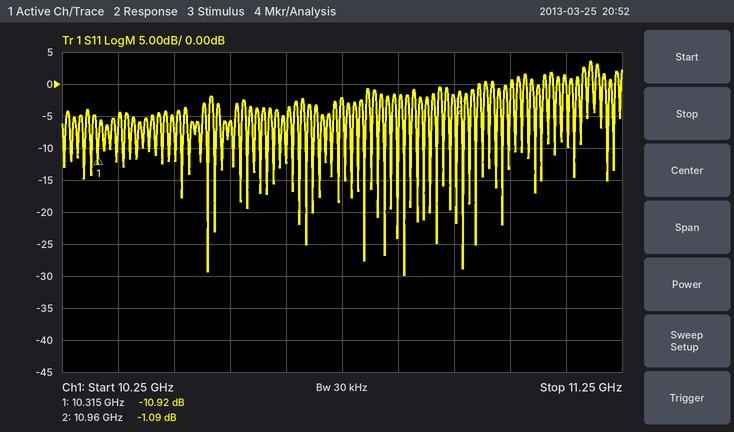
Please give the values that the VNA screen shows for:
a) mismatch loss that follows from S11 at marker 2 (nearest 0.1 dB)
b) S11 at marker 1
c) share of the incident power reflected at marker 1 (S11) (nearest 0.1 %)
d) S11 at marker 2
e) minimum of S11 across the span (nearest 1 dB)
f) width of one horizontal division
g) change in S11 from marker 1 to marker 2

6.5 dB
-10.92 dB
8.1 %
-1.09 dB
-30 dB
100 MHz
9.83 dB
